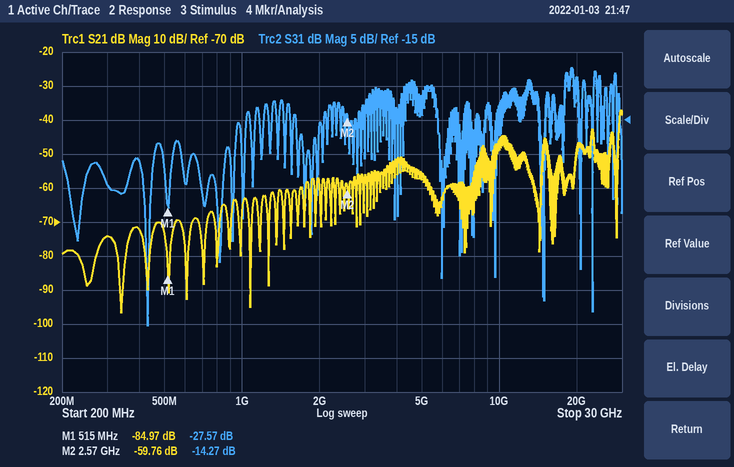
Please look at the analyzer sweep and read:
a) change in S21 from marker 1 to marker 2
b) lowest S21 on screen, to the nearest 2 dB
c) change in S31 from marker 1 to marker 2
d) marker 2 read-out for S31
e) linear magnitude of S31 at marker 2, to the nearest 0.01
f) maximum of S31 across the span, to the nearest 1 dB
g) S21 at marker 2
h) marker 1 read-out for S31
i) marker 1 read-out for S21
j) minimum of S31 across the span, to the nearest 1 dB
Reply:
25.21 dB
-96 dB
13.30 dB
-14.27 dB
0.19
-7 dB
-59.76 dB
-27.57 dB
-84.97 dB
-45 dB
